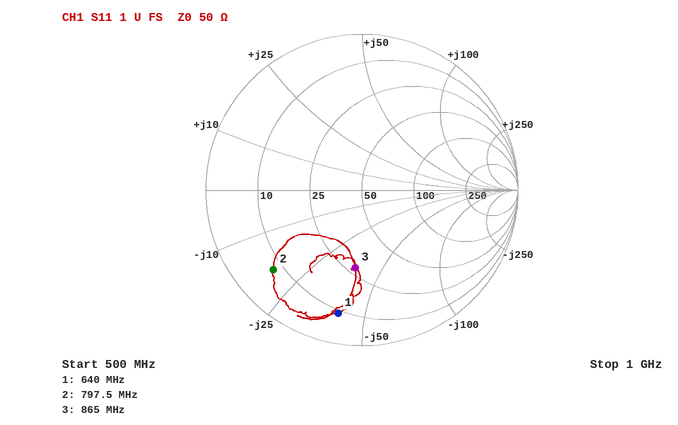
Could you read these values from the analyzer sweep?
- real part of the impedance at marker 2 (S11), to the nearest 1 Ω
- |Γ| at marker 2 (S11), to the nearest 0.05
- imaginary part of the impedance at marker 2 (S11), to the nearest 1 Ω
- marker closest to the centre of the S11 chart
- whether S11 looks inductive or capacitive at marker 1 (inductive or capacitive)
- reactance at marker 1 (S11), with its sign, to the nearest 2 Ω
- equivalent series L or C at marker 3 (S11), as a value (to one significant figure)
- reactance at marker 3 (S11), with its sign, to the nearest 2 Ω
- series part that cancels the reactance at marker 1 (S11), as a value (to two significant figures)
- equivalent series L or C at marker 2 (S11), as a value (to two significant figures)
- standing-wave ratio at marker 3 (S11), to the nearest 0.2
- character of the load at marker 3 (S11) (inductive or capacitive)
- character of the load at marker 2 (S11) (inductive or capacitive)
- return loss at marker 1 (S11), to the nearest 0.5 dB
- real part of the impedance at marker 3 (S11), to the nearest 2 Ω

8 Ω
0.75
-19 Ω
marker 3
capacitive
-40 Ω
5 pF
-38 Ω
10 nH
11 pF
3.0
capacitive
capacitive
2.0 dB
28 Ω
